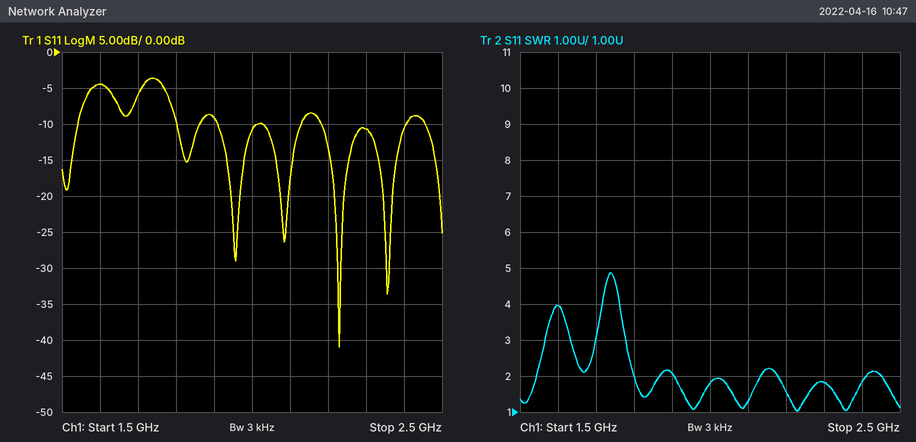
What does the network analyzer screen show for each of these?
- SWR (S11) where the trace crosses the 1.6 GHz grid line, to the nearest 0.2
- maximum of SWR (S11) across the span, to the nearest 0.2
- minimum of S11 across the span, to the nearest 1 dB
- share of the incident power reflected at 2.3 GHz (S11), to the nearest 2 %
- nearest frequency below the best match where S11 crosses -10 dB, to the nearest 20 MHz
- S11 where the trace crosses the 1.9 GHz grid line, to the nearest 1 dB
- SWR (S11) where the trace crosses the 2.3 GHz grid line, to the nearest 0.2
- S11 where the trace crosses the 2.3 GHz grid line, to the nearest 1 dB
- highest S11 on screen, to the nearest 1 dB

4.0
4.8
-41 dB
8 %
2.18 GHz
-9 dB
1.8
-11 dB
-4 dB
